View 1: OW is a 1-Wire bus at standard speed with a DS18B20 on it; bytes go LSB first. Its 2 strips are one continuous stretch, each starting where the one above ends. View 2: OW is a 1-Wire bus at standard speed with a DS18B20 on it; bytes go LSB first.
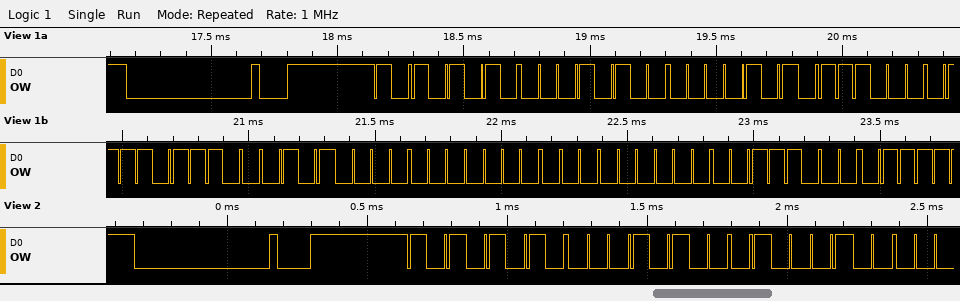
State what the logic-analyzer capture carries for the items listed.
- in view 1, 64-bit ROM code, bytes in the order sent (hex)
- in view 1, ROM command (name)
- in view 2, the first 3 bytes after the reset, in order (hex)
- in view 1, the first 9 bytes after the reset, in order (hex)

28 50 87 3B 0A 00 00 1C
Match ROM
55 28 22
55 28 50 87 3B 0A 00 00 1C
